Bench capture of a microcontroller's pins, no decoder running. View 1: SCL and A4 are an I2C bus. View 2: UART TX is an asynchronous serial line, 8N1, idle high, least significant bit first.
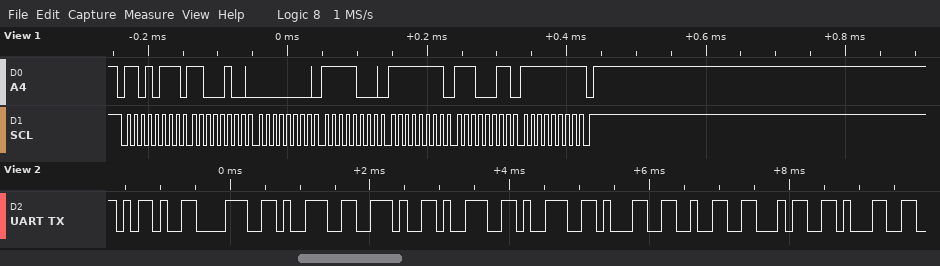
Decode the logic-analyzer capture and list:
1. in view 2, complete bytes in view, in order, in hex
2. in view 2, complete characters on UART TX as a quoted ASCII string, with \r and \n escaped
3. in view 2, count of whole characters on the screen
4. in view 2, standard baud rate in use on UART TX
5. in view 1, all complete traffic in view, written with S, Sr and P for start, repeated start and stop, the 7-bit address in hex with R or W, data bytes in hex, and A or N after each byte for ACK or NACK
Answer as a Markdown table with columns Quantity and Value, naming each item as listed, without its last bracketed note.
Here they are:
| Quantity | Value |
|---|---|
| in view 2, complete bytes in view, in order, in hex | 2D 38 39 2E 39 39 31 32 34 31 |
| in view 2, complete characters on UART TX as a quoted ASCII string, with \r and \n escaped | "-89.991241" |
| in view 2, count of whole characters on the screen | 10 |
| in view 2, standard baud rate in use on UART TX | 9600 baud |
| in view 1, all complete traffic in view, written with S, Sr and P for start, repeated start and stop, the 7-bit address in hex with R or W, data bytes in hex, and A or N after each byte for ACK or NACK | S 6BR A C4 A 00 A F8 A FF A E3 A FF N P |
